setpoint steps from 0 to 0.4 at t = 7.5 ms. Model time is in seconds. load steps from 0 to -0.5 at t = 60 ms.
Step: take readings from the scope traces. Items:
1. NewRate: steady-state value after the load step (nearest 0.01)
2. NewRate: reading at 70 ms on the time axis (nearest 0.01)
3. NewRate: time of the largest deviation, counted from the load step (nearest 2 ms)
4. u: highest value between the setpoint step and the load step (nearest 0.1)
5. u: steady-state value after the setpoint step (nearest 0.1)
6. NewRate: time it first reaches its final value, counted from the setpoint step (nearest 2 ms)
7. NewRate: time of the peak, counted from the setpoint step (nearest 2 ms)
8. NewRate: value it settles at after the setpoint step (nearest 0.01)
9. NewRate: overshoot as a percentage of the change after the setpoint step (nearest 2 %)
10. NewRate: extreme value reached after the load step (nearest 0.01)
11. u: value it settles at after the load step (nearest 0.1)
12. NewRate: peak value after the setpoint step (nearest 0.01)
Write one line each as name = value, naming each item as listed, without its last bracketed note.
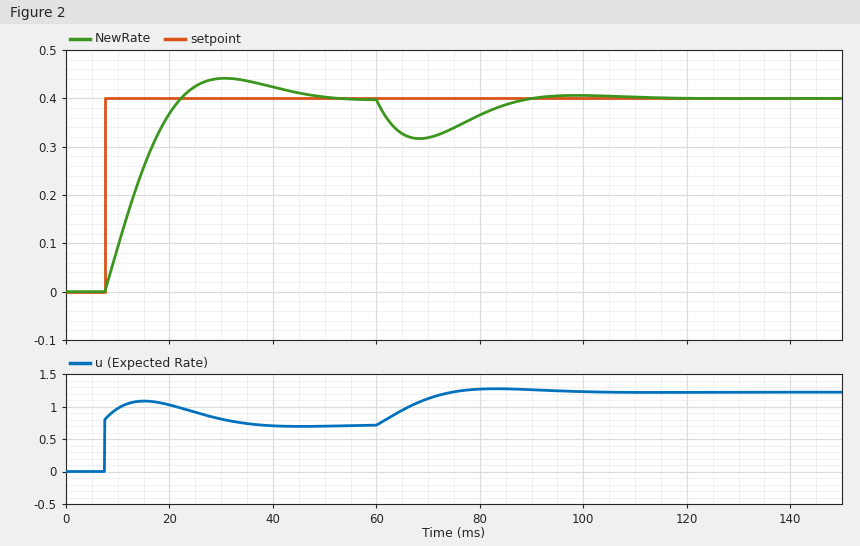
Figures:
NewRate: steady-state value after the load step = 0.40
NewRate: reading at 70 ms on the time axis = 0.32
NewRate: time of the largest deviation, counted from the load step = 8 ms
u: highest value between the setpoint step and the load step = 1.1
u: steady-state value after the setpoint step = 0.7
NewRate: time it first reaches its final value, counted from the setpoint step = 14 ms
NewRate: time of the peak, counted from the setpoint step = 24 ms
NewRate: value it settles at after the setpoint step = 0.40
NewRate: overshoot as a percentage of the change after the setpoint step = 10 %
NewRate: extreme value reached after the load step = 0.32
u: value it settles at after the load step = 1.2
NewRate: peak value after the setpoint step = 0.44
